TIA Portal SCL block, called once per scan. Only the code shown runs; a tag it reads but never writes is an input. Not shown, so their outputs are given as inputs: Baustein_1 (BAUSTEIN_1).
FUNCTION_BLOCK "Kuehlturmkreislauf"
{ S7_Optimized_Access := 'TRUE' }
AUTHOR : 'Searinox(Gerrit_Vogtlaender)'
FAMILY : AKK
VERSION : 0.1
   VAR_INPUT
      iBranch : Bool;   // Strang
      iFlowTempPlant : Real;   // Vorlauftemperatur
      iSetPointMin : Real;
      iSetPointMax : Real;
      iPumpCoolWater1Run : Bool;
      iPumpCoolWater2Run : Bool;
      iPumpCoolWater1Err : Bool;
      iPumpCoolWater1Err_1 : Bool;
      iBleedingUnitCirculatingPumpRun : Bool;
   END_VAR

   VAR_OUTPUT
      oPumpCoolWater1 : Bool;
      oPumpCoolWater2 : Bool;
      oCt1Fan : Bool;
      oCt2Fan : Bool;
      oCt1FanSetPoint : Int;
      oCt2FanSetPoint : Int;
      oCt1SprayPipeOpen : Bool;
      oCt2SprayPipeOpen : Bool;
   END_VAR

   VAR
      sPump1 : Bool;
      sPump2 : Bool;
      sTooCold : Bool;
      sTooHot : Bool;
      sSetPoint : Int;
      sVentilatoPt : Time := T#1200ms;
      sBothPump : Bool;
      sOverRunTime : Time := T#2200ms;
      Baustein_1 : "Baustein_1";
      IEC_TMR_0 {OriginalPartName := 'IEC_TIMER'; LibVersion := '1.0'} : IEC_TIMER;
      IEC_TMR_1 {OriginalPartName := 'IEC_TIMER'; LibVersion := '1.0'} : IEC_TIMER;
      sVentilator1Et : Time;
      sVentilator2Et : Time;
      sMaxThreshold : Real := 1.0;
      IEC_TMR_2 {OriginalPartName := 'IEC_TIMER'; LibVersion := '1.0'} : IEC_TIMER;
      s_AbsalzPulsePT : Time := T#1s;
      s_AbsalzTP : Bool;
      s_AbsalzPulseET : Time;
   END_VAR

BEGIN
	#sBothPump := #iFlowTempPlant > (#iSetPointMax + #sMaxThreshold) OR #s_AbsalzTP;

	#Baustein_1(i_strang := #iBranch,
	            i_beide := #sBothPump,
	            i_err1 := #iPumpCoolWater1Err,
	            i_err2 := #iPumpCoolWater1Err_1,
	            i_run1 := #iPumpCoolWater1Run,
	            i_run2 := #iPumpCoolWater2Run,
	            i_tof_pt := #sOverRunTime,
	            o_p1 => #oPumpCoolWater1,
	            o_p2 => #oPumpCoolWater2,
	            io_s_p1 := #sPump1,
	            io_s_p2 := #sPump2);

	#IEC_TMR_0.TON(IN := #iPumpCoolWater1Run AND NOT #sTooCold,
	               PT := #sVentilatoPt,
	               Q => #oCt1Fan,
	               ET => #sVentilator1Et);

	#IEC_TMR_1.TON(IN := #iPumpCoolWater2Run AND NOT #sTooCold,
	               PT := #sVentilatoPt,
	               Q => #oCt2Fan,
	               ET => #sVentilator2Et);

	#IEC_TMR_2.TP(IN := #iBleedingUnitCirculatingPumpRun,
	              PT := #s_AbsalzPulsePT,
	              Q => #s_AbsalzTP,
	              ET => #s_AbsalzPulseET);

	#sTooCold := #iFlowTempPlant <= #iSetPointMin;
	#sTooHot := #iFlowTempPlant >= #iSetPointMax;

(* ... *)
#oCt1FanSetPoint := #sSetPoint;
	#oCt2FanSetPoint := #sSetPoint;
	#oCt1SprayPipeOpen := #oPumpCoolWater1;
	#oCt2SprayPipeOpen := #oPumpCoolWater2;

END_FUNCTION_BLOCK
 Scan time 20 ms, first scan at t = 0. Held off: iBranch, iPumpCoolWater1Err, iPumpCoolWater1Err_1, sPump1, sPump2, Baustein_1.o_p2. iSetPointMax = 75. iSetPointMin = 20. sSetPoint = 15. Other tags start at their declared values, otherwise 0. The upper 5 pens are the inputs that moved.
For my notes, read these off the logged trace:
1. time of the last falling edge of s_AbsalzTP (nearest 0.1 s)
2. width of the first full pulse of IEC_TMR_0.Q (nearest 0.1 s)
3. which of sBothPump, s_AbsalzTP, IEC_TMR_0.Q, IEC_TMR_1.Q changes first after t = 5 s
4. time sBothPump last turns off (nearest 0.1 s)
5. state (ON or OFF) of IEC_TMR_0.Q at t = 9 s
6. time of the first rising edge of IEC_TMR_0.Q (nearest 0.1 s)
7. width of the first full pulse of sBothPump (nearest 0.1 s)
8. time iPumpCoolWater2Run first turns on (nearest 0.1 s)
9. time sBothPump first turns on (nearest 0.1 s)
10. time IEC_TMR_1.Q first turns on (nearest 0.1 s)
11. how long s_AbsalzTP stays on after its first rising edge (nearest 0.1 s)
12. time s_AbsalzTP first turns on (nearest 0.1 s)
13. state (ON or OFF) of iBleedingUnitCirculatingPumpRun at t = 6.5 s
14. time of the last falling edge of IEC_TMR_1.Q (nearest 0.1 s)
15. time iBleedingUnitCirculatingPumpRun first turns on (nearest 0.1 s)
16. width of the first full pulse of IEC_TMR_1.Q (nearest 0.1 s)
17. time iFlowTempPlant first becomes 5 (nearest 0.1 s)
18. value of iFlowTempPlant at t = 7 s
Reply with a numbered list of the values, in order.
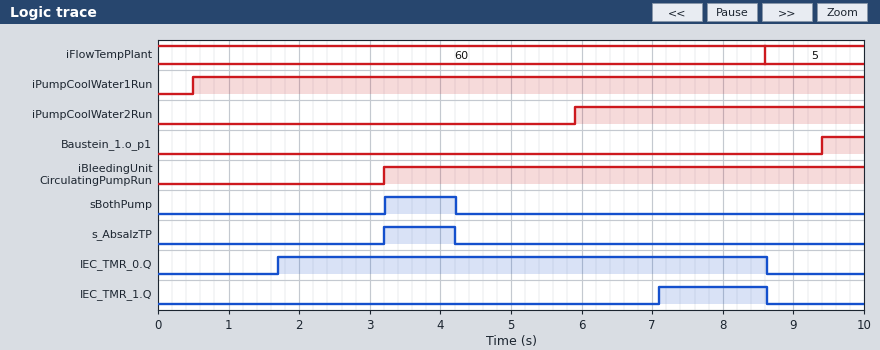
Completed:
1. 4.2 s
2. 6.9 s
3. IEC_TMR_1.Q
4. 4.2 s
5. OFF
6. 1.7 s
7. 1.0 s
8. 5.9 s
9. 3.2 s
10. 7.1 s
11. 1.0 s
12. 3.2 s
13. ON
14. 8.6 s
15. 3.2 s
16. 1.5 s
17. 8.6 s
18. 60
